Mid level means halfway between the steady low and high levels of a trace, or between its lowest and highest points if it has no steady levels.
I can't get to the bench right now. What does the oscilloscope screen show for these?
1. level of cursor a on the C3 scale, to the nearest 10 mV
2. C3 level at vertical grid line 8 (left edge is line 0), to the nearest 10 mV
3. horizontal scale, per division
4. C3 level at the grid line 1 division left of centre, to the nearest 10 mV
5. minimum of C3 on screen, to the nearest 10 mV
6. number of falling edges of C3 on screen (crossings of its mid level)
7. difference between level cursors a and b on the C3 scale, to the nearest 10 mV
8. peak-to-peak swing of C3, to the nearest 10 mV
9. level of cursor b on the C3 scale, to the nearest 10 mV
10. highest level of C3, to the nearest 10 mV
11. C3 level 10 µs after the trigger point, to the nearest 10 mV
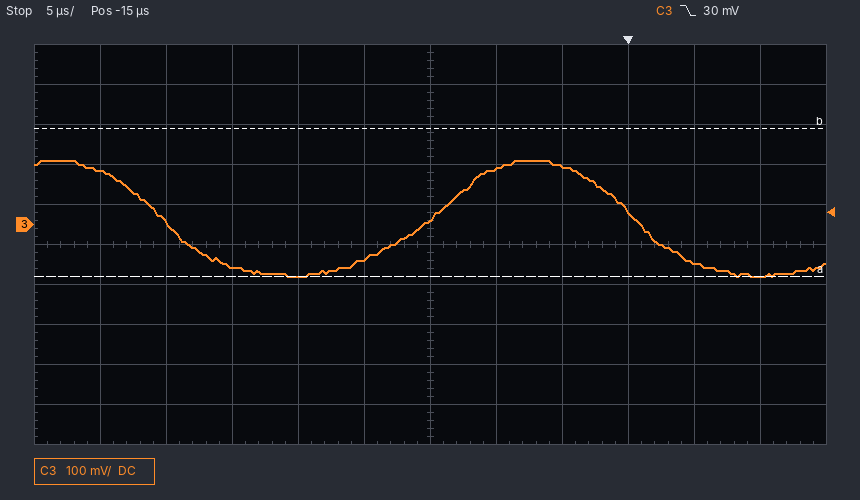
-130 mV
150 mV
5 µs
-90 mV
-130 mV
2
370 mV
290 mV
240 mV
160 mV
-130 mV
